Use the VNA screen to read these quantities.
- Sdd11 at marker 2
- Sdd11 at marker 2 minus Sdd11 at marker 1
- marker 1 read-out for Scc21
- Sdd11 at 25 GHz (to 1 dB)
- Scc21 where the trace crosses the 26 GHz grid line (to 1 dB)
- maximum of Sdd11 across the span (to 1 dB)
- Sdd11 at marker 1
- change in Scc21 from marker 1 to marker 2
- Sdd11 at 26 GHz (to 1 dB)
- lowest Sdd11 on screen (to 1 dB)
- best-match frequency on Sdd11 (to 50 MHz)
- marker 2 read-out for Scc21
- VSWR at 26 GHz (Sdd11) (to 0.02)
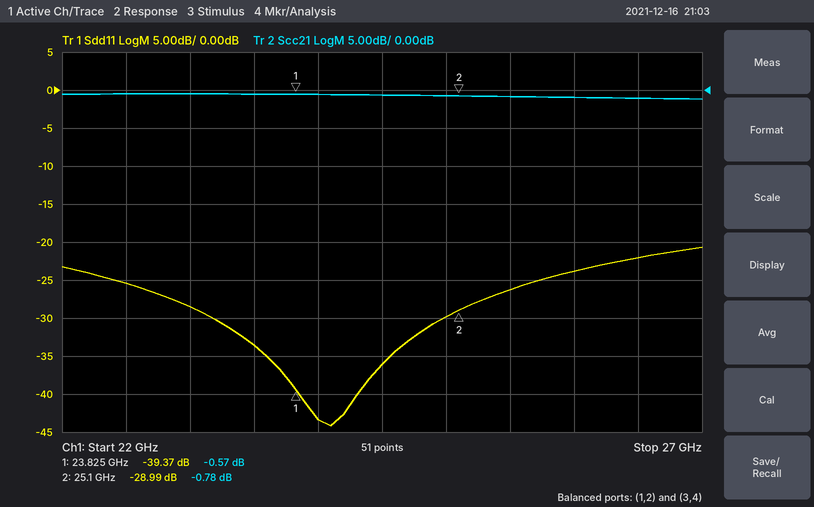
-28.99 dB
10.38 dB
-0.57 dB
-30 dB
-1 dB
-21 dB
-39.37 dB
-0.21 dB
-24 dB
-44 dB
24.10 GHz
-0.78 dB
1.14
